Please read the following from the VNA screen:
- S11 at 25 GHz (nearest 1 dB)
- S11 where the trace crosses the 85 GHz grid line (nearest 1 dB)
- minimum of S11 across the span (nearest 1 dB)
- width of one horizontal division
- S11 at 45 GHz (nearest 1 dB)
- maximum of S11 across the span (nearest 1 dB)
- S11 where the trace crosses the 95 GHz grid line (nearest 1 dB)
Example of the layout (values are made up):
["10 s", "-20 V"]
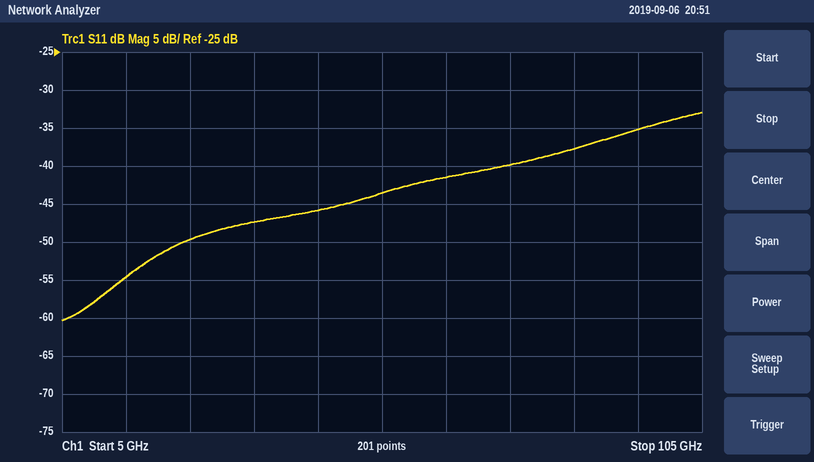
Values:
["-50 dB", "-38 dB", "-60 dB", "10 GHz", "-46 dB", "-33 dB", "-35 dB"]
